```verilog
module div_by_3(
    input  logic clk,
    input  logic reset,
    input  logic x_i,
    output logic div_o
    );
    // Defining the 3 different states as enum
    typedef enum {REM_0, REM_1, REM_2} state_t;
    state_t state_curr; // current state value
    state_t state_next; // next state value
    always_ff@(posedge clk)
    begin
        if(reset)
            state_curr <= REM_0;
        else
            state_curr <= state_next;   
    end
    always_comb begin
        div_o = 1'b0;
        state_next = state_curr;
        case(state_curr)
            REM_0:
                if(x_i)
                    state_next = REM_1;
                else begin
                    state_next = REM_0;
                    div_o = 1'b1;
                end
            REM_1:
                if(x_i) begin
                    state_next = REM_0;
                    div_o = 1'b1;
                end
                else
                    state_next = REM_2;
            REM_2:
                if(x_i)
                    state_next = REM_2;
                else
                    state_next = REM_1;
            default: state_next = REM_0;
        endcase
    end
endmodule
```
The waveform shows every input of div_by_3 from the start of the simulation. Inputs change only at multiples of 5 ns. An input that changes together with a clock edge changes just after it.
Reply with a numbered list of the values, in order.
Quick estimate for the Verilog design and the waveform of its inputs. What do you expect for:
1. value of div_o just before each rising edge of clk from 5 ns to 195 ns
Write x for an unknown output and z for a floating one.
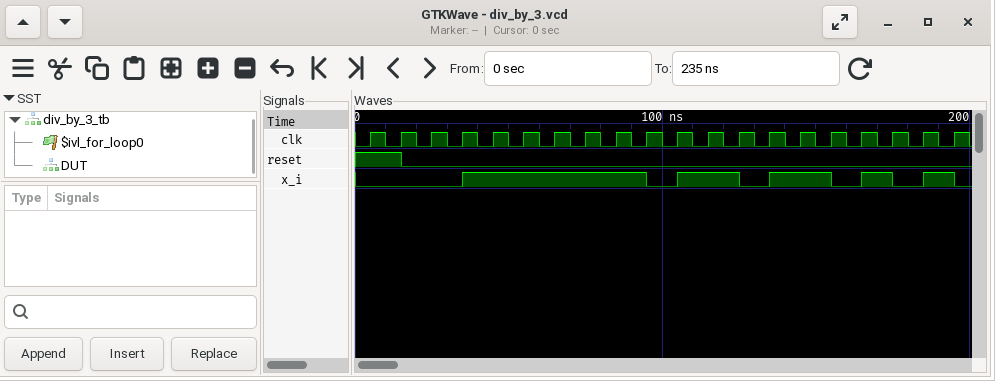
1. 1 1 1 1 0 1 0 1 0 1 1 0 1 1 0 1 1 0 0 0
